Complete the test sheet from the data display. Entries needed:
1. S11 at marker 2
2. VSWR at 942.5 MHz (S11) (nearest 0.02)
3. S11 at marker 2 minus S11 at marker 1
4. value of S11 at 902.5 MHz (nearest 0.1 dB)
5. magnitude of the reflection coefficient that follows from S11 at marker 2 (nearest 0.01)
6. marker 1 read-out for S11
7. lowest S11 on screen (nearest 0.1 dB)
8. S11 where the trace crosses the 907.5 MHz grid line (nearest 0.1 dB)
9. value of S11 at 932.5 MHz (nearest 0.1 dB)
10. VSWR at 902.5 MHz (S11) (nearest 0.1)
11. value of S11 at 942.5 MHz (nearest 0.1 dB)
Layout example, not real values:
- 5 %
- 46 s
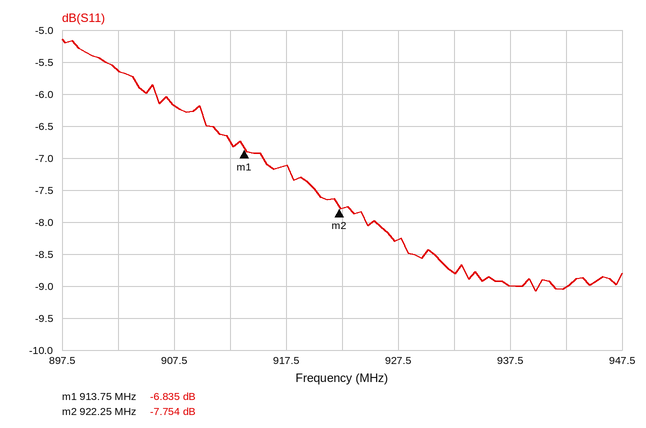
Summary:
- -7.754 dB
- 2.10
- -0.919 dB
- -5.6 dB
- 0.41
- -6.835 dB
- -9.1 dB
- -6.2 dB
- -8.8 dB
- 3.2
- -9.0 dB
